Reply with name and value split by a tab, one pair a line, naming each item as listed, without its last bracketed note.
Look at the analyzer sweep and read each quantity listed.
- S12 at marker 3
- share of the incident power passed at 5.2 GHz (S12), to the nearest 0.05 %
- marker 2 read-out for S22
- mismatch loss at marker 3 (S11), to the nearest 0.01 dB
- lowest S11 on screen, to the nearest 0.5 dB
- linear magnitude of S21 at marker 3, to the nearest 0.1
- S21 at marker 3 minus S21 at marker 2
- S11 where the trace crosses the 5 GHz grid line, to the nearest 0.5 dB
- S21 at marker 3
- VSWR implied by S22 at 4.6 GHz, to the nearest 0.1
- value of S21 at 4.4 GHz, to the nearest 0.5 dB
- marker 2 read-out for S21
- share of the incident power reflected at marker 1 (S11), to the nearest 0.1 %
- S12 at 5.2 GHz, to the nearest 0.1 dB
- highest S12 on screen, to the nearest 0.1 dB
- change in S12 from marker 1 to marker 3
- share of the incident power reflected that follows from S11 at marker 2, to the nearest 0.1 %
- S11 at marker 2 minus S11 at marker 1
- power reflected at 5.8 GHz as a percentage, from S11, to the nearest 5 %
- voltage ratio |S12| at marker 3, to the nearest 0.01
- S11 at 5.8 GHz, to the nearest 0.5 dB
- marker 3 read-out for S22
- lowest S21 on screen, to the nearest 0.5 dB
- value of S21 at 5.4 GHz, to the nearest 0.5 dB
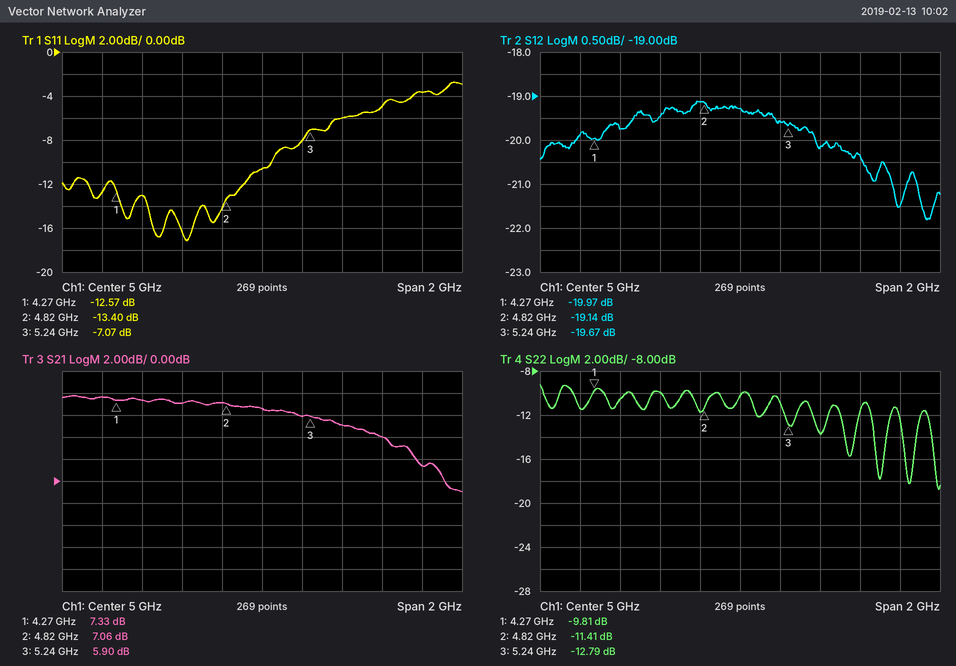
S12 at marker 3	-19.67 dB
share of the incident power passed at 5.2 GHz (S12), to the nearest 0.05 %	1.10 %
marker 2 read-out for S22	-11.41 dB
mismatch loss at marker 3 (S11), to the nearest 0.01 dB	0.95 dB
lowest S11 on screen, to the nearest 0.5 dB	-17.0 dB
linear magnitude of S21 at marker 3, to the nearest 0.1	2.0
S21 at marker 3 minus S21 at marker 2	-1.16 dB
S11 where the trace crosses the 5 GHz grid line, to the nearest 0.5 dB	-10.5 dB
S21 at marker 3	5.90 dB
VSWR implied by S22 at 4.6 GHz, to the nearest 0.1	1.9
value of S21 at 4.4 GHz, to the nearest 0.5 dB	7.5 dB
marker 2 read-out for S21	7.06 dB
share of the incident power reflected at marker 1 (S11), to the nearest 0.1 %	5.5 %
S12 at 5.2 GHz, to the nearest 0.1 dB	-19.6 dB
highest S12 on screen, to the nearest 0.1 dB	-19.1 dB
change in S12 from marker 1 to marker 3	0.30 dB
share of the incident power reflected that follows from S11 at marker 2, to the nearest 0.1 %	4.6 %
S11 at marker 2 minus S11 at marker 1	-0.83 dB
power reflected at 5.8 GHz as a percentage, from S11, to the nearest 5 %	45 %
voltage ratio |S12| at marker 3, to the nearest 0.01	0.10
S11 at 5.8 GHz, to the nearest 0.5 dB	-3.5 dB
marker 3 read-out for S22	-12.79 dB
lowest S21 on screen, to the nearest 0.5 dB	-1.0 dB
value of S21 at 5.4 GHz, to the nearest 0.5 dB	5.0 dB
